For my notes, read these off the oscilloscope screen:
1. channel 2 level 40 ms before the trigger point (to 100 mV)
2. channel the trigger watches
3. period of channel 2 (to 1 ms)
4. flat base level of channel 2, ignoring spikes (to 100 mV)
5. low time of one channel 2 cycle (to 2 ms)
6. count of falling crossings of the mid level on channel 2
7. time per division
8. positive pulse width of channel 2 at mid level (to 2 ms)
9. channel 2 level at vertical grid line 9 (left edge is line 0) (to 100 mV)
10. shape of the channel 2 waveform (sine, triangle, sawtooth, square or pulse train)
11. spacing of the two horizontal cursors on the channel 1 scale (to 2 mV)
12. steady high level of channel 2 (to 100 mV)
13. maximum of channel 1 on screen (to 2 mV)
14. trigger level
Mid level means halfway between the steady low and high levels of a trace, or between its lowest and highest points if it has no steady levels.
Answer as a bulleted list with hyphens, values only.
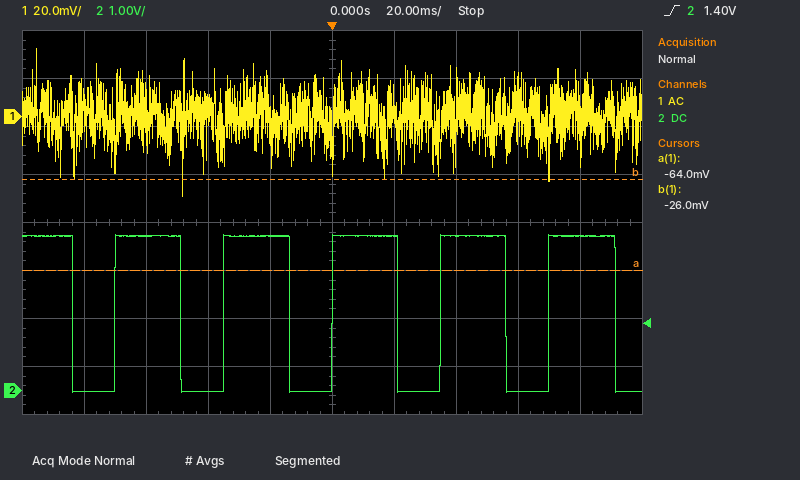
- 0.0 V
- channel 2
- 35 ms
- 0.0 V
- 14 ms
- 6
- 20 ms
- 22 ms
- 3.2 V
- pulse train
- 38 mV
- 3.2 V
- 28 mV
- 1.40 V
